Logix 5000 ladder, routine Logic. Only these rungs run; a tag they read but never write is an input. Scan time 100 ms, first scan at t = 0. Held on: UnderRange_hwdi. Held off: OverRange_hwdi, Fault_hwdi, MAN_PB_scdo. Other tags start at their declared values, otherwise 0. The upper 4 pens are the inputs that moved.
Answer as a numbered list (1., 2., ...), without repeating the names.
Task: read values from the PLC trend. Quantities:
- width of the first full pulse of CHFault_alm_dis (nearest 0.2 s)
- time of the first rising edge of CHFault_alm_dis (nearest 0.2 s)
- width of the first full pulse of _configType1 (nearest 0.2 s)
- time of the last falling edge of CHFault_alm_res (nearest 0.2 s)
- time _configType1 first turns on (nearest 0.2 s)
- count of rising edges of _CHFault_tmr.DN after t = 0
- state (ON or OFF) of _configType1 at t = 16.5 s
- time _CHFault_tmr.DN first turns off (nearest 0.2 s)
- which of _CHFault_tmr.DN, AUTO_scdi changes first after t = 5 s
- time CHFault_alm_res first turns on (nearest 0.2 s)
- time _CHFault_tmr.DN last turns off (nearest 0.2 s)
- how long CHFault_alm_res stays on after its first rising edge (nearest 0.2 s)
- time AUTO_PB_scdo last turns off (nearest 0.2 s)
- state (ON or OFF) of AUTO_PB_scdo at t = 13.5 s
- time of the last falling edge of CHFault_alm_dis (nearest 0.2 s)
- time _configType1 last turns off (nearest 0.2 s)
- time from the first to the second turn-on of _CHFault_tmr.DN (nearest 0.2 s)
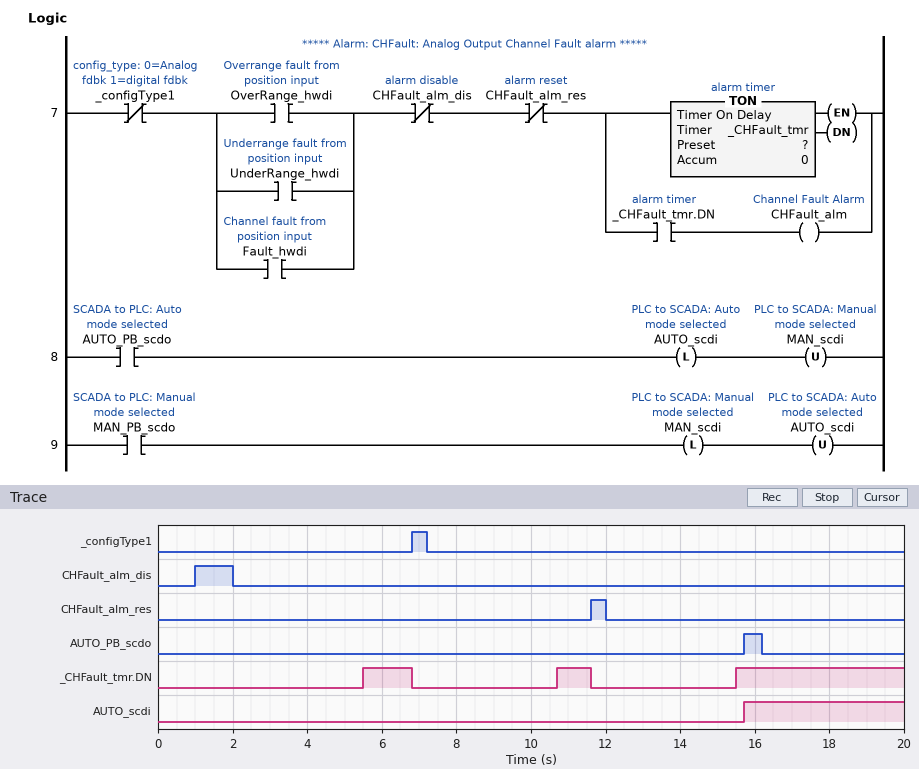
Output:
1. 1.0 s
2. 1.0 s
3. 0.4 s
4. 12.0 s
5. 6.8 s
6. 3
7. OFF
8. 6.8 s
9. _CHFault_tmr.DN
10. 11.6 s
11. 11.6 s
12. 0.4 s
13. 16.2 s
14. OFF
15. 2.0 s
16. 7.2 s
17. 5.2 s
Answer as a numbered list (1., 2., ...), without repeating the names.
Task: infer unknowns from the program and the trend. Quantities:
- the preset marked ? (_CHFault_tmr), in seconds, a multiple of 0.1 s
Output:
1. 3.5 s
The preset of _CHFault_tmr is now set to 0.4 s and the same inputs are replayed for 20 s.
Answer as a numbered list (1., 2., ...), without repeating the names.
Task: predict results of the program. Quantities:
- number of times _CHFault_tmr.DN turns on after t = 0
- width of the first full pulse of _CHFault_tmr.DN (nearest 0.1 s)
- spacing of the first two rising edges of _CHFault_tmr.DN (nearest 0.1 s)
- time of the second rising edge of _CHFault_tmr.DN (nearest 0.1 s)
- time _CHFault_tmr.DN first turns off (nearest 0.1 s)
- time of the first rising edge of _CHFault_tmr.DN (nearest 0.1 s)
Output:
1. 4
2. 0.6 s
3. 2.0 s
4. 2.4 s
5. 1.0 s
6. 0.4 s
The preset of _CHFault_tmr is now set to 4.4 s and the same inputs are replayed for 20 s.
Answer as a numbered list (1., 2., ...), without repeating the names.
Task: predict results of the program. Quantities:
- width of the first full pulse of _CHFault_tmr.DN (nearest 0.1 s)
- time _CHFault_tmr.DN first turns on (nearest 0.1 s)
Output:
1. 0.4 s
2. 6.4 s
